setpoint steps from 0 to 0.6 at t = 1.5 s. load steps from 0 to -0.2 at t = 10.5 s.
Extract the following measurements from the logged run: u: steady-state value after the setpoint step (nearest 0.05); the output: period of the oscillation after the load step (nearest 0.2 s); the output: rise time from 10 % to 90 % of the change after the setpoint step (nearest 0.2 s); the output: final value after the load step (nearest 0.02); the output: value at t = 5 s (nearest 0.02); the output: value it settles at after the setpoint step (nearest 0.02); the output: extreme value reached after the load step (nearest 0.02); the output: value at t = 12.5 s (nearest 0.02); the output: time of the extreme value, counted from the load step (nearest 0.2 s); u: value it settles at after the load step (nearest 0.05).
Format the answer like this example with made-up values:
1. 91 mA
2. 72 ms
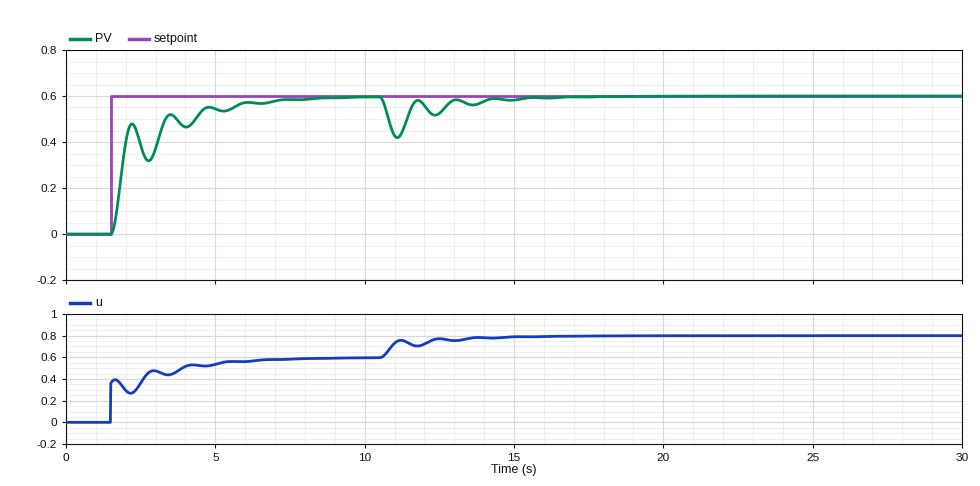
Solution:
1. 0.60
2. 1.2 s
3. 3.0 s
4. 0.60
5. 0.54
6. 0.60
7. 0.42
8. 0.52
9. 0.6 s
10. 0.80
